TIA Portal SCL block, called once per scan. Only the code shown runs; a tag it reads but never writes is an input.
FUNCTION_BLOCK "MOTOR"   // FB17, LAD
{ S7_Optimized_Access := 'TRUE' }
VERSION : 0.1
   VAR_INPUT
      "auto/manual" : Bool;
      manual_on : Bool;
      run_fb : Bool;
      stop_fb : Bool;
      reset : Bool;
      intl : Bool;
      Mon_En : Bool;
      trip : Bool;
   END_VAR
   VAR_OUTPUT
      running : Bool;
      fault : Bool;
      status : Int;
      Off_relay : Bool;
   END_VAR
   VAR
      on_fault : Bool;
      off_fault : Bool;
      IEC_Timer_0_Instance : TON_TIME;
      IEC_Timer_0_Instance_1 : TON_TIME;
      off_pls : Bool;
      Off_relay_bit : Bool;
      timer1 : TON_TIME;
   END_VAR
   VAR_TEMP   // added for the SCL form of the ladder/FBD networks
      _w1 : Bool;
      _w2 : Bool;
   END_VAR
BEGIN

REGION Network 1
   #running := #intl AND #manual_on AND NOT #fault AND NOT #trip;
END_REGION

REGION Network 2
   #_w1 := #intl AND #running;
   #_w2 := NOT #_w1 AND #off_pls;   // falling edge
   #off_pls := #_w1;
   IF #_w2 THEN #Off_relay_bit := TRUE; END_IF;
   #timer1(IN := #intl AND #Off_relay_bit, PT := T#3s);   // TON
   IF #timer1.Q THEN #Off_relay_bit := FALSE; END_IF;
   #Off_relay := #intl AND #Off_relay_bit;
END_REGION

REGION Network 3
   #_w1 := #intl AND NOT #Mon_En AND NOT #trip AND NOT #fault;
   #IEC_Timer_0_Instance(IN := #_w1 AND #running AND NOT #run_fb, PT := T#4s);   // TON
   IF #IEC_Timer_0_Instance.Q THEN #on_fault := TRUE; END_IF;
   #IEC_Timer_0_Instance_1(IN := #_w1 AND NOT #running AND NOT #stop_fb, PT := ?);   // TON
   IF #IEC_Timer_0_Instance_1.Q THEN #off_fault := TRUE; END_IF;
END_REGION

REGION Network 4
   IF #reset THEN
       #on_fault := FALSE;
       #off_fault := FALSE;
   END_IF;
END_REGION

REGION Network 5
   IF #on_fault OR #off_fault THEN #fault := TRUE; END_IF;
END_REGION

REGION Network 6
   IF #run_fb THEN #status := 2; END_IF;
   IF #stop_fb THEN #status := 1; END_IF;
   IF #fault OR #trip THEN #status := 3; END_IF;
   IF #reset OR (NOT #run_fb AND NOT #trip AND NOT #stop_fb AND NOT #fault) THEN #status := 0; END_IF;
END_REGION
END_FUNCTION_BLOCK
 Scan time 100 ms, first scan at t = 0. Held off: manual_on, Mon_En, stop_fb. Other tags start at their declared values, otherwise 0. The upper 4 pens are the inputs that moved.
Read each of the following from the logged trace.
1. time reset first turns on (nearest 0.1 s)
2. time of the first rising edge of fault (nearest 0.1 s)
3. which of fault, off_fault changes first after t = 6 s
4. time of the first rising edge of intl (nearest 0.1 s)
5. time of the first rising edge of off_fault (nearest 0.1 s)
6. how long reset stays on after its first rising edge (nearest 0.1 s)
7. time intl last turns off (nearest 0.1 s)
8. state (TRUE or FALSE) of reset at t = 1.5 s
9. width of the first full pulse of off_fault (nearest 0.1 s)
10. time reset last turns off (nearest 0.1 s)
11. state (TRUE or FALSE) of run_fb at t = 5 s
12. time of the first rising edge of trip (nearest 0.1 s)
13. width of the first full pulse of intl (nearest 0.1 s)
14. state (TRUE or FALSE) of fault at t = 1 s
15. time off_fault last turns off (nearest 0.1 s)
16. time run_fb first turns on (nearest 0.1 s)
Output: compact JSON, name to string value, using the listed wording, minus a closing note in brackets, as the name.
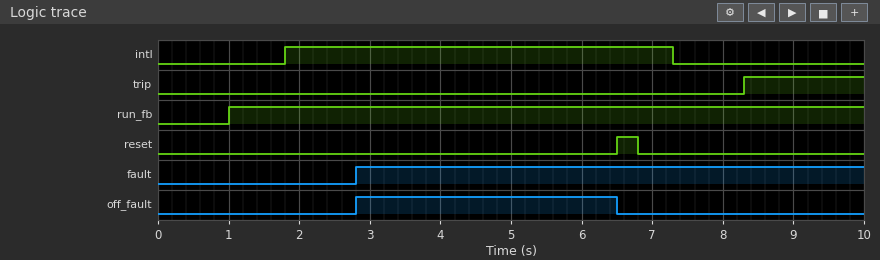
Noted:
{"time reset first turns on": "6.5 s", "time of the first rising edge of fault": "2.8 s", "which of fault, off_fault changes first after t = 6 s": "off_fault", "time of the first rising edge of intl": "1.8 s", "time of the first rising edge of off_fault": "2.8 s", "how long reset stays on after its first rising edge": "0.3 s", "time intl last turns off": "7.3 s", "state (TRUE or FALSE) of reset at t = 1.5 s": "FALSE", "width of the first full pulse of off_fault": "3.7 s", "time reset last turns off": "6.8 s", "state (TRUE or FALSE) of run_fb at t = 5 s": "TRUE", "time of the first rising edge of trip": "8.3 s", "width of the first full pulse of intl": "5.5 s", "state (TRUE or FALSE) of fault at t = 1 s": "FALSE", "time off_fault last turns off": "6.5 s", "time run_fb first turns on": "1.0 s"}
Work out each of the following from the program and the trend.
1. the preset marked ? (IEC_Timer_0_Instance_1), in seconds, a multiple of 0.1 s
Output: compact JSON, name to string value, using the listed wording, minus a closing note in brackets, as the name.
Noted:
{"the preset marked ? (IEC_Timer_0_Instance_1), in seconds, a multiple of 0.1 s": "1.0 s"}
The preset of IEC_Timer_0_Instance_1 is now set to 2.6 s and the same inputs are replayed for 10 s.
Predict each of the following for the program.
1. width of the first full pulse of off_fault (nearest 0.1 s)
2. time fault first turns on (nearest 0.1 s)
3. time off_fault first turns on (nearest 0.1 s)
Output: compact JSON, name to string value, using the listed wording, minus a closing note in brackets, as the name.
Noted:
{"width of the first full pulse of off_fault": "2.1 s", "time fault first turns on": "4.4 s", "time off_fault first turns on": "4.4 s"}
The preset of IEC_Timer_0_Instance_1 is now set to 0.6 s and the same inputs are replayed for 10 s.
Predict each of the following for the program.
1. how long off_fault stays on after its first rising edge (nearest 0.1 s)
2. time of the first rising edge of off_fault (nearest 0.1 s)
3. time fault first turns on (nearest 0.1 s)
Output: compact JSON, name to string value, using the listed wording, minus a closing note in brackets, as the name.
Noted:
{"how long off_fault stays on after its first rising edge": "4.1 s", "time of the first rising edge of off_fault": "2.4 s", "time fault first turns on": "2.4 s"}
